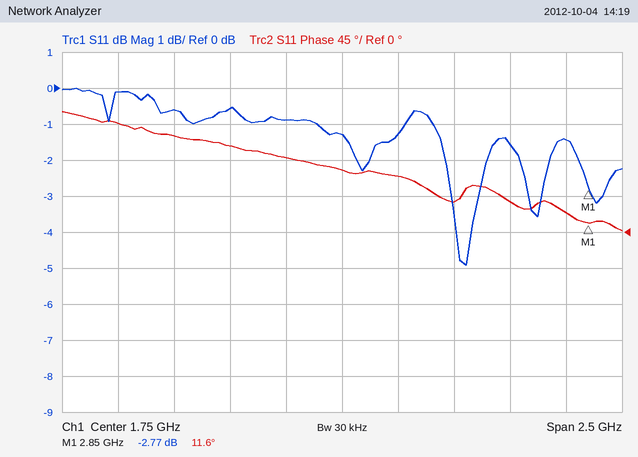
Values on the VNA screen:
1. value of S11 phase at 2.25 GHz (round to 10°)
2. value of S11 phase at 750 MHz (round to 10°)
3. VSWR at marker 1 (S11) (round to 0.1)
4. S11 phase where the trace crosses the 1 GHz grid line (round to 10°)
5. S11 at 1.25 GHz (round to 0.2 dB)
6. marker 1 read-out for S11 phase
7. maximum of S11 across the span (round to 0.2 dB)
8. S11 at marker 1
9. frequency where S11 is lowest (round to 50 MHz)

40°
140°
6.3
120°
-0.6 dB
11.6°
0.0 dB
-2.77 dB
2.30 GHz
